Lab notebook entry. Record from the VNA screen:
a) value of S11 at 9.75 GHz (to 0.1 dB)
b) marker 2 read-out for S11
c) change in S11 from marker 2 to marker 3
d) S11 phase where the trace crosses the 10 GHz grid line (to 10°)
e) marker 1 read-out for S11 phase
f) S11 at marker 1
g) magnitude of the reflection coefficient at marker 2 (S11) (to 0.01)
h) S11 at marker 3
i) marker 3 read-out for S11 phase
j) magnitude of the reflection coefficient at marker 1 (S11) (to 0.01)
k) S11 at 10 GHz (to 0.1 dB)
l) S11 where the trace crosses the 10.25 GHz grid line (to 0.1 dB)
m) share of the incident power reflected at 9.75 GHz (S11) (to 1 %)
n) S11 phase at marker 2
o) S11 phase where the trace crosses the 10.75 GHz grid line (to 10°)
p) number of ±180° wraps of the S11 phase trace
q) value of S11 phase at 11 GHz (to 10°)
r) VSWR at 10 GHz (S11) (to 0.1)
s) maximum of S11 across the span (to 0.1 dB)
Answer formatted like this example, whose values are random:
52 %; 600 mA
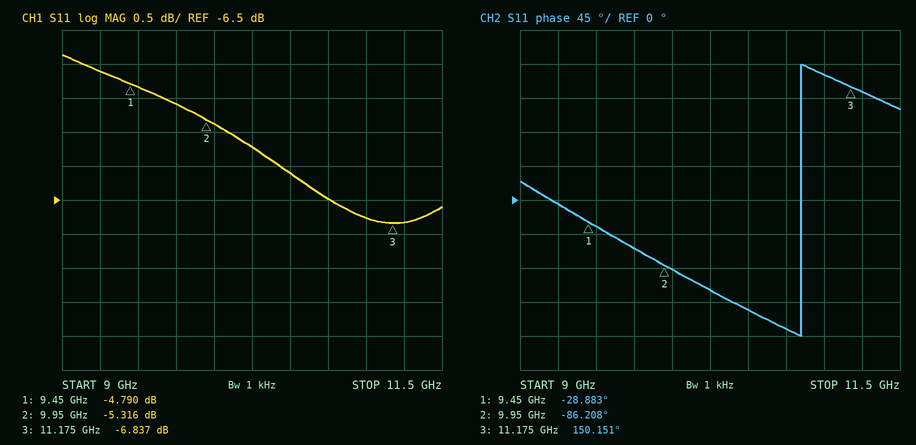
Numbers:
-5.1 dB; -5.316 dB; -1.521 dB; -90°; -28.883°; -4.790 dB; 0.54; -6.837 dB; 150.151°; 0.58; -5.4 dB; -5.7 dB; 31 %; -86.208°; -170°; 1; 170°; 3.3; -4.4 dB
